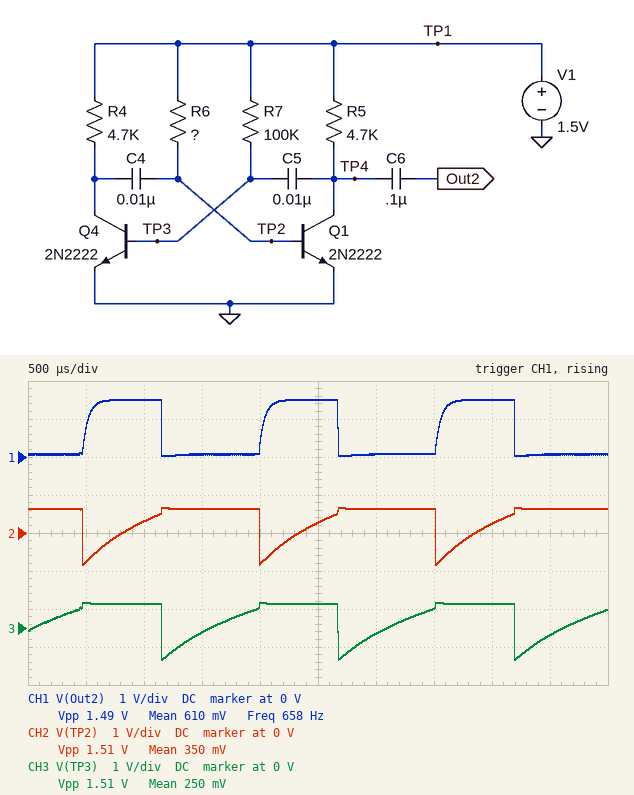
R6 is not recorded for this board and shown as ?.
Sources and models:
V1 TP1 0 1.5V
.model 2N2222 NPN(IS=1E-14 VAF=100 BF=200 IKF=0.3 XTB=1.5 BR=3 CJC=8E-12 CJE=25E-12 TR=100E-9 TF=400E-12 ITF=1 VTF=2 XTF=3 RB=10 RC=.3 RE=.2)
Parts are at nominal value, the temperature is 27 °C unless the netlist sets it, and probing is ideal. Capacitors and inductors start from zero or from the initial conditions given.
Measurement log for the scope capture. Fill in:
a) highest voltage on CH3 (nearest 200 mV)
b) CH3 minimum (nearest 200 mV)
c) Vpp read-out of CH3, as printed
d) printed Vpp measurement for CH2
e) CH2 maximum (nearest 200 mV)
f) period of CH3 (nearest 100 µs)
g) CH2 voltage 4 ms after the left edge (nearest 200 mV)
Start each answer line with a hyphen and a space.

- 600 mV
- -800 mV
- 1.51 V
- 1.51 V
- 600 mV
- 1.5 ms
- 200 mV
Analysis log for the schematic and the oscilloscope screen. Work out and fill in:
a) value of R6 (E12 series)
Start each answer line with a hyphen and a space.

- 82 kΩ
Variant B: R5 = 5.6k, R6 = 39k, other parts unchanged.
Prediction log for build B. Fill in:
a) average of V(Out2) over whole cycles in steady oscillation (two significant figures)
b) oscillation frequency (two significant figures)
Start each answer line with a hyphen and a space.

- 370 mV
- 840 Hz
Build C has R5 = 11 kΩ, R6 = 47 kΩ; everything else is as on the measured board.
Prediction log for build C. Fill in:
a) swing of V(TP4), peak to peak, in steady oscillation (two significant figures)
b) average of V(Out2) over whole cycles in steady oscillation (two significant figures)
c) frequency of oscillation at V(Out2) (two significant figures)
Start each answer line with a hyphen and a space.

- 1.4 V
- 380 mV
- 800 Hz
